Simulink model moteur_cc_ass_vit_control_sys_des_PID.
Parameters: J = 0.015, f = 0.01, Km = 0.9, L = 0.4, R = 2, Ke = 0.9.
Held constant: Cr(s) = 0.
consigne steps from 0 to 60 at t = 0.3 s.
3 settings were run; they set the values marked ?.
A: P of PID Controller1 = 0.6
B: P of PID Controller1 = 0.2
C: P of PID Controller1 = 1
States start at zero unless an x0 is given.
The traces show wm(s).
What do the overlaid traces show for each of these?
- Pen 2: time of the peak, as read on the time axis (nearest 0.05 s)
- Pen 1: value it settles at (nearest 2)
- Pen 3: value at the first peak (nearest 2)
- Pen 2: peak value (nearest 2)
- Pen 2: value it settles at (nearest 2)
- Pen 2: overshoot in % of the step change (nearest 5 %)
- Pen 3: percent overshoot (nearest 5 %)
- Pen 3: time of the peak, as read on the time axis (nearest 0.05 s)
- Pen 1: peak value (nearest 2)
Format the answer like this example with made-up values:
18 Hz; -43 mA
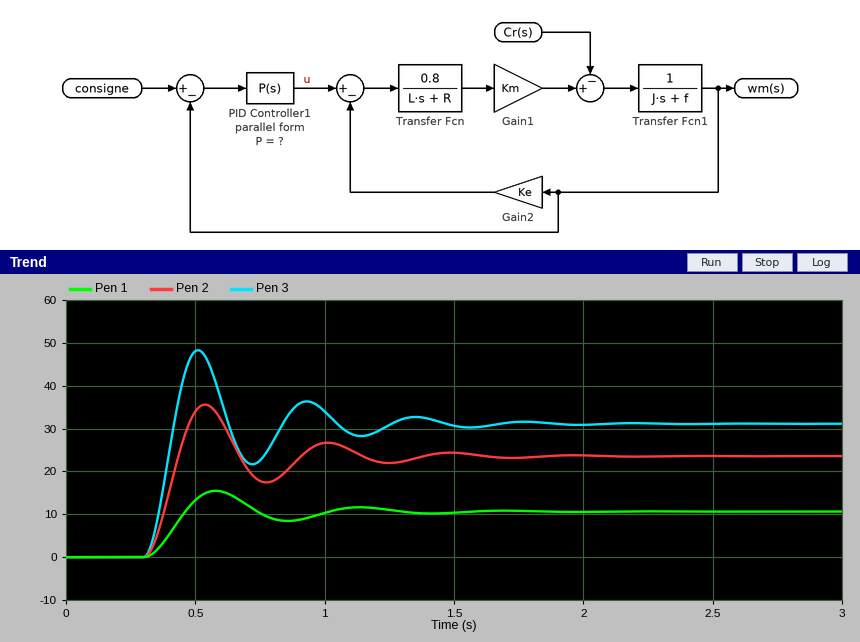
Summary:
0.55 s; 10; 48; 36; 24; 50 %; 55 %; 0.50 s; 16
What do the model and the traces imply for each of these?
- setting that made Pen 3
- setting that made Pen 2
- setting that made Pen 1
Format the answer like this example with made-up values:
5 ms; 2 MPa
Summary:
C; A; B
